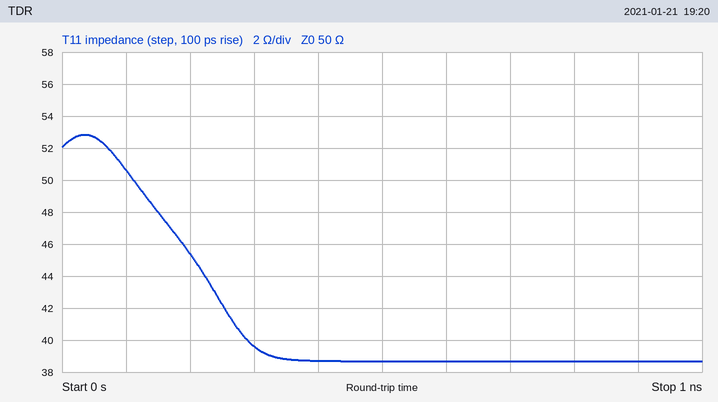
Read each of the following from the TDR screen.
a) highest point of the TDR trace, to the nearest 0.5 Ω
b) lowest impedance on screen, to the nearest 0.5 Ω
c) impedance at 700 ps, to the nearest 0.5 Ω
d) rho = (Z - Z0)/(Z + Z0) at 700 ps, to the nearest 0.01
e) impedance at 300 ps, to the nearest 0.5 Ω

53.0 Ω
38.5 Ω
38.5 Ω
-0.13
39.5 Ω
